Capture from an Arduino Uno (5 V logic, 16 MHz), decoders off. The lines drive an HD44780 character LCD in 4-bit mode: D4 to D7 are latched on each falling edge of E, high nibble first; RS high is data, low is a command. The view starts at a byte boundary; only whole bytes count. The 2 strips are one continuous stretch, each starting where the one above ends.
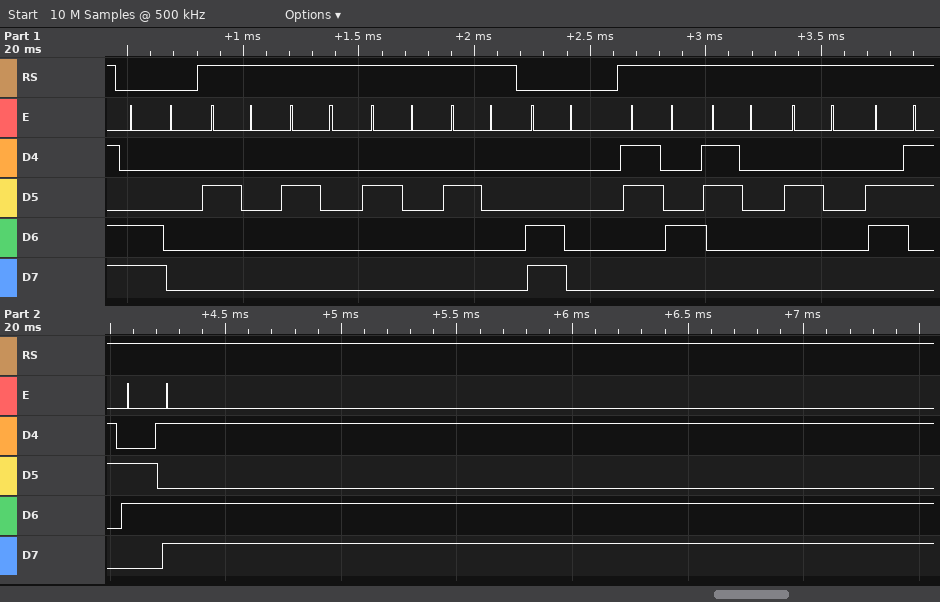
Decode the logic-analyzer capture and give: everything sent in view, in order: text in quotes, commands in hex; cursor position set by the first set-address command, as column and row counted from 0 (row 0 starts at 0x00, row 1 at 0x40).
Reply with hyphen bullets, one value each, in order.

- 0xC0 "    " 0xC0 "40 cm"
- column 0, row 1
